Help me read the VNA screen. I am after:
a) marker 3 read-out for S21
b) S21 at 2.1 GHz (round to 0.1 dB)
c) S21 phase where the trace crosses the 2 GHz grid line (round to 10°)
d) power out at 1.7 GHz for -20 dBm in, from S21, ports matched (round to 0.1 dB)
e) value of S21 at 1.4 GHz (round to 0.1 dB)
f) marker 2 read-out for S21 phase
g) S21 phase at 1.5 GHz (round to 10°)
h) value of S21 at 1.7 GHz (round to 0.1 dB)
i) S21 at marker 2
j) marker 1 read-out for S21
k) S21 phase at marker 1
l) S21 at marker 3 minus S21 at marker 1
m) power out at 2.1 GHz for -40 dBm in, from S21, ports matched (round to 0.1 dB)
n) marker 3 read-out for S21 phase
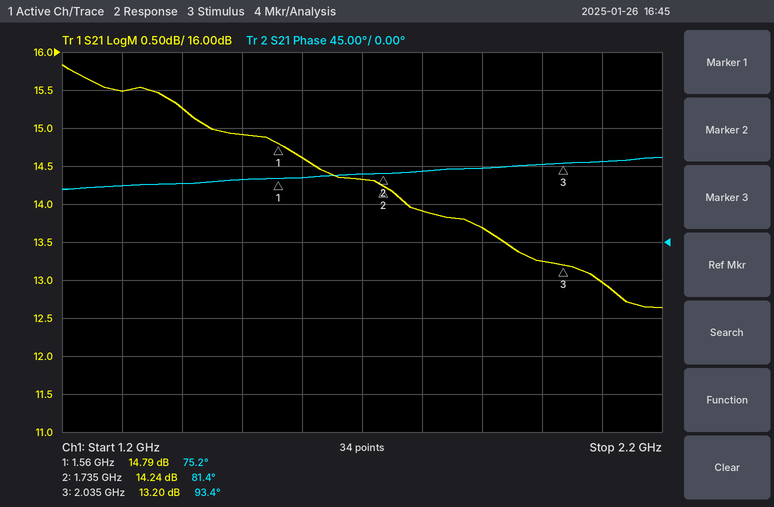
13.20 dB
13.0 dB
90°
-5.7 dBm
15.3 dB
81.4°
70°
14.3 dB
14.24 dB
14.79 dB
75.2°
-1.59 dB
-27.0 dBm
93.4°
